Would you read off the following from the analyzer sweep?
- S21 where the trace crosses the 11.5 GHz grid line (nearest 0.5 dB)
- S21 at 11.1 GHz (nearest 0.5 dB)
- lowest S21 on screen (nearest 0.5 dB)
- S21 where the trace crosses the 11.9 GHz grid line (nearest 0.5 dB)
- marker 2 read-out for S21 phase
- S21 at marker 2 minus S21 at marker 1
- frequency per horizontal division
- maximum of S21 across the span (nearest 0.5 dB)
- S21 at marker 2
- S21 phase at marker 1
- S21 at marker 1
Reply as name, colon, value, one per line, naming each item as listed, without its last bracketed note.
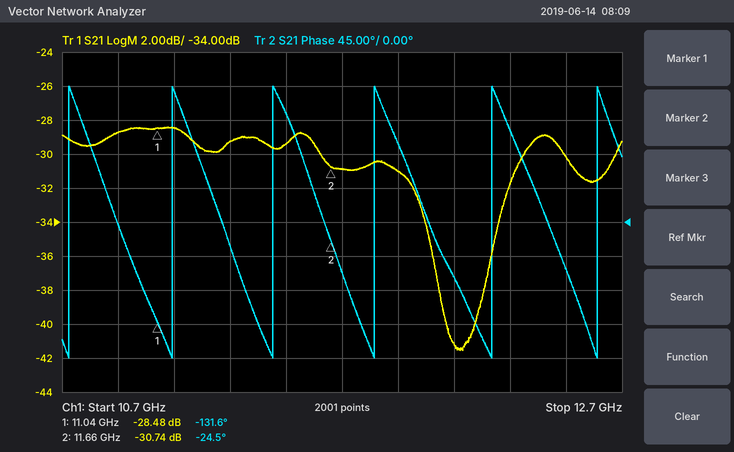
S21 where the trace crosses the 11.5 GHz grid line: -29.5 dB
S21 at 11.1 GHz: -28.5 dB
lowest S21 on screen: -41.5 dB
S21 where the trace crosses the 11.9 GHz grid line: -31.0 dB
marker 2 read-out for S21 phase: -24.5°
S21 at marker 2 minus S21 at marker 1: -2.26 dB
frequency per horizontal division: 200 MHz
maximum of S21 across the span: -28.5 dB
S21 at marker 2: -30.74 dB
S21 phase at marker 1: -131.6°
S21 at marker 1: -28.48 dB
